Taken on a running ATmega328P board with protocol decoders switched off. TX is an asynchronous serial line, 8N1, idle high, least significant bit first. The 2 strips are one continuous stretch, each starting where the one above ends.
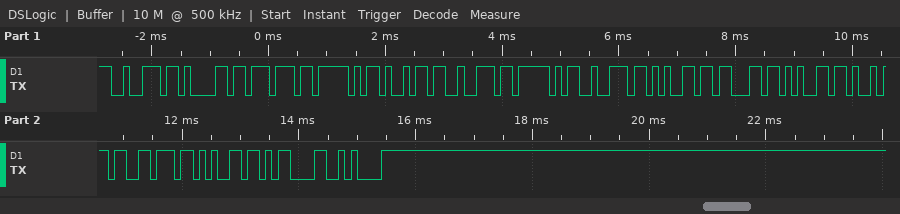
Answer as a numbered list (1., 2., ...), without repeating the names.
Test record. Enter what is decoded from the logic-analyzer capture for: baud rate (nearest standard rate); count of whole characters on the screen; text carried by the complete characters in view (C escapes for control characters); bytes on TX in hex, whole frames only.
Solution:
1. 9600 baud
2. 16
3. "raw_ir_receive\r\n"
4. 72 61 77 5F 69 72 5F 72 65 63 65 69 76 65 0D 0A
